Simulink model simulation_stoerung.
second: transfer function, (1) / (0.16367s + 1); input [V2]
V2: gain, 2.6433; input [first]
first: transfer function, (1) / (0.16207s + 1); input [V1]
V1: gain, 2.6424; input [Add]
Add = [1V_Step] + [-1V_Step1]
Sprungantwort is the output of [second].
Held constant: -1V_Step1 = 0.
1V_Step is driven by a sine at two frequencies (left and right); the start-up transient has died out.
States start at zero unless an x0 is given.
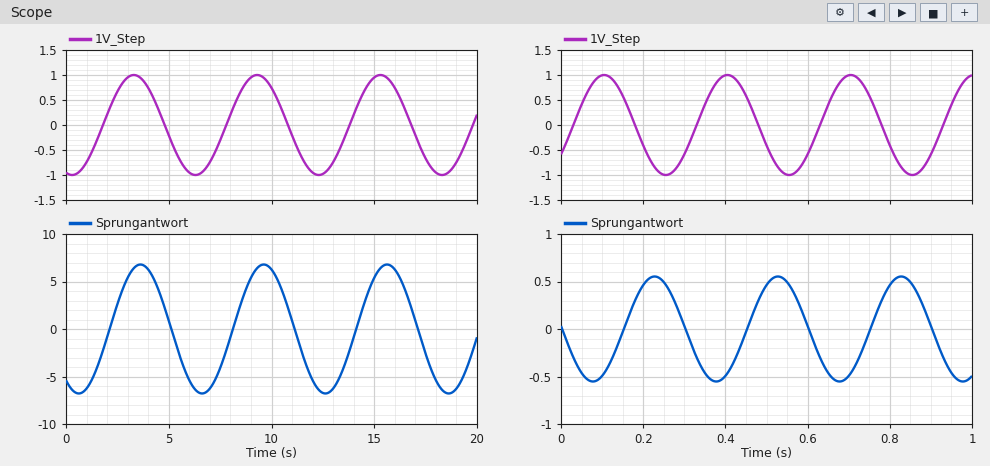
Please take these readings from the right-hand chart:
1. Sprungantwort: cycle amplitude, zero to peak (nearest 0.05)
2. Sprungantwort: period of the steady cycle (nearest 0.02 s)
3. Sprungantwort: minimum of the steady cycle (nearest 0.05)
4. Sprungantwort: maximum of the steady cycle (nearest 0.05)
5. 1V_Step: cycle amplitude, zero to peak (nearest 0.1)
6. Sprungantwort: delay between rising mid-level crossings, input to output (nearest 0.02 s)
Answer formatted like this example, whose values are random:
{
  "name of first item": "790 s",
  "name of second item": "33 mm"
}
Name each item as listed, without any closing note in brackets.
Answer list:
{
  "Sprungantwort: cycle amplitude, zero to peak": "0.55",
  "Sprungantwort: period of the steady cycle": "0.30 s",
  "Sprungantwort: minimum of the steady cycle": "-0.55",
  "Sprungantwort: maximum of the steady cycle": "0.55",
  "1V_Step: cycle amplitude, zero to peak": "1.0",
  "Sprungantwort: delay between rising mid-level crossings, input to output": "0.12 s"
}
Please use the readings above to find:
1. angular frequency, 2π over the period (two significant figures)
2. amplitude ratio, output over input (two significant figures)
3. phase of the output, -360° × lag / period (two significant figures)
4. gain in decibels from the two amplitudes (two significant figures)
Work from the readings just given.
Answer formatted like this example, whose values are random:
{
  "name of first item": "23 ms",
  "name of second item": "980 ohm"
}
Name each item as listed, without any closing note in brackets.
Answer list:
{
  "angular frequency, 2π over the period": "21 rad/s",
  "amplitude ratio, output over input": "0.55",
  "phase of the output, -360° × lag / period": "-140°",
  "gain in decibels from the two amplitudes": "-5.2 dB"
}
